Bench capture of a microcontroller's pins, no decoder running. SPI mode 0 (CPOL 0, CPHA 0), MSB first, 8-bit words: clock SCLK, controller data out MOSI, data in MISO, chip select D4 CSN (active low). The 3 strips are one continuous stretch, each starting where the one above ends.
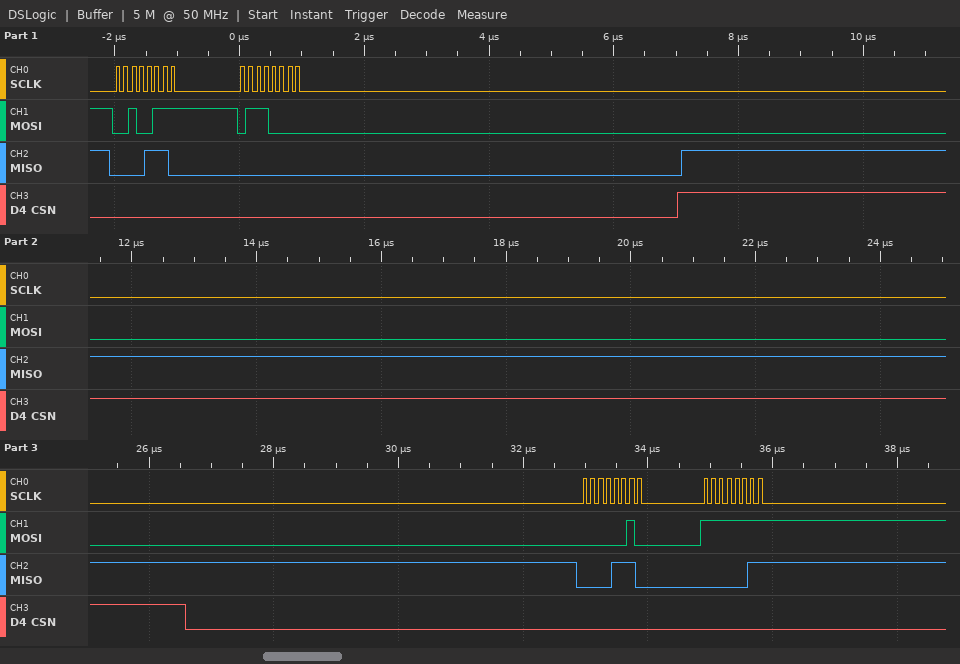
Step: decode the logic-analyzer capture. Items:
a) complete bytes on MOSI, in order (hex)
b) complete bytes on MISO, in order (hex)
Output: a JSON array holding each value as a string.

["27 70 02 FF", "0E 00 0E 03"]
